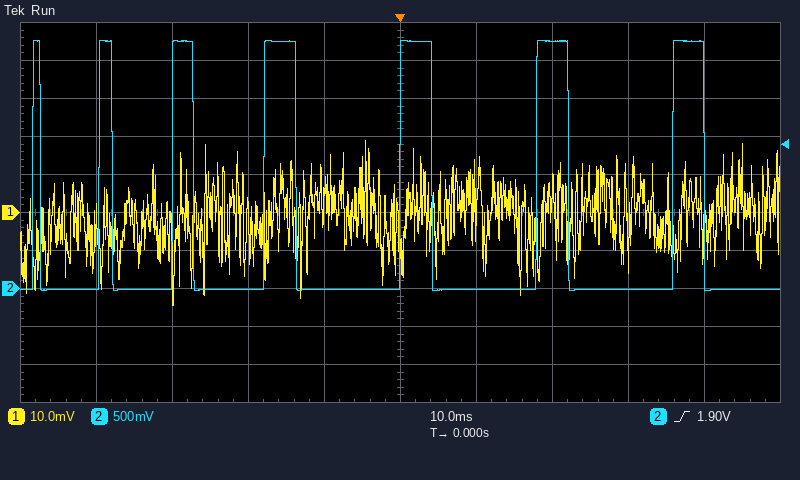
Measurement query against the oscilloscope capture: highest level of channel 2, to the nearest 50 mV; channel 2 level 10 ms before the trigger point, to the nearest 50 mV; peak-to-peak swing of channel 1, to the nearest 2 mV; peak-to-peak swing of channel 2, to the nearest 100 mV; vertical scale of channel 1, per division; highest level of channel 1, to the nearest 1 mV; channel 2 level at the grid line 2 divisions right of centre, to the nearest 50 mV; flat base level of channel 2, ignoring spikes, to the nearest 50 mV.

3.25 V
0 mV
44 mV
3.30 V
10 mV
19 mV
3.25 V
0 mV
